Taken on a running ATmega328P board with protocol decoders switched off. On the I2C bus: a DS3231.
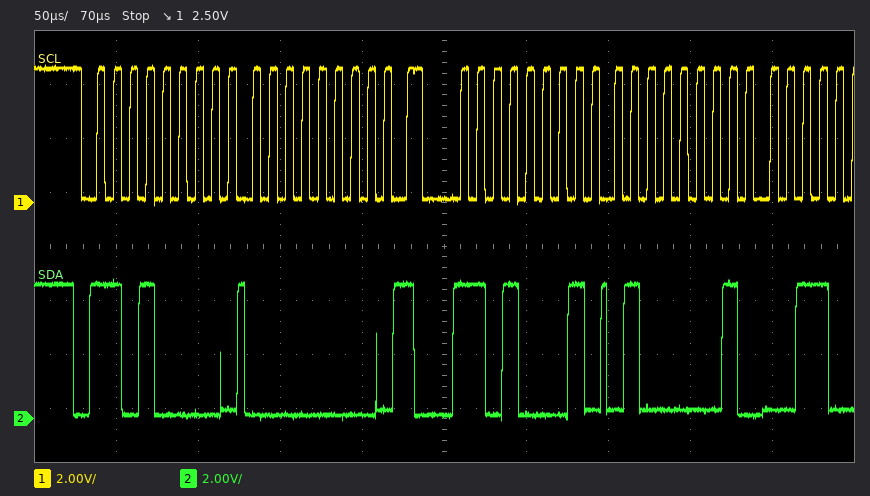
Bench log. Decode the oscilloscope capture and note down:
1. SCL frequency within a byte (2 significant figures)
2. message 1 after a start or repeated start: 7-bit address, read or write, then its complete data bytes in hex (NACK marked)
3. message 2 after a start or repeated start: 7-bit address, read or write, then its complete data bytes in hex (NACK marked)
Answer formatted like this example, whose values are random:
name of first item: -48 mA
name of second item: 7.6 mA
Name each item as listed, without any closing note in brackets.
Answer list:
SCL frequency within a byte: 100 kHz
message 1 after a start or repeated start: 7-bit address, read or write, then its complete data bytes in hex: 0x68 write: 00
message 2 after a start or repeated start: 7-bit address, read or write, then its complete data bytes in hex: 0x68 read: 41
